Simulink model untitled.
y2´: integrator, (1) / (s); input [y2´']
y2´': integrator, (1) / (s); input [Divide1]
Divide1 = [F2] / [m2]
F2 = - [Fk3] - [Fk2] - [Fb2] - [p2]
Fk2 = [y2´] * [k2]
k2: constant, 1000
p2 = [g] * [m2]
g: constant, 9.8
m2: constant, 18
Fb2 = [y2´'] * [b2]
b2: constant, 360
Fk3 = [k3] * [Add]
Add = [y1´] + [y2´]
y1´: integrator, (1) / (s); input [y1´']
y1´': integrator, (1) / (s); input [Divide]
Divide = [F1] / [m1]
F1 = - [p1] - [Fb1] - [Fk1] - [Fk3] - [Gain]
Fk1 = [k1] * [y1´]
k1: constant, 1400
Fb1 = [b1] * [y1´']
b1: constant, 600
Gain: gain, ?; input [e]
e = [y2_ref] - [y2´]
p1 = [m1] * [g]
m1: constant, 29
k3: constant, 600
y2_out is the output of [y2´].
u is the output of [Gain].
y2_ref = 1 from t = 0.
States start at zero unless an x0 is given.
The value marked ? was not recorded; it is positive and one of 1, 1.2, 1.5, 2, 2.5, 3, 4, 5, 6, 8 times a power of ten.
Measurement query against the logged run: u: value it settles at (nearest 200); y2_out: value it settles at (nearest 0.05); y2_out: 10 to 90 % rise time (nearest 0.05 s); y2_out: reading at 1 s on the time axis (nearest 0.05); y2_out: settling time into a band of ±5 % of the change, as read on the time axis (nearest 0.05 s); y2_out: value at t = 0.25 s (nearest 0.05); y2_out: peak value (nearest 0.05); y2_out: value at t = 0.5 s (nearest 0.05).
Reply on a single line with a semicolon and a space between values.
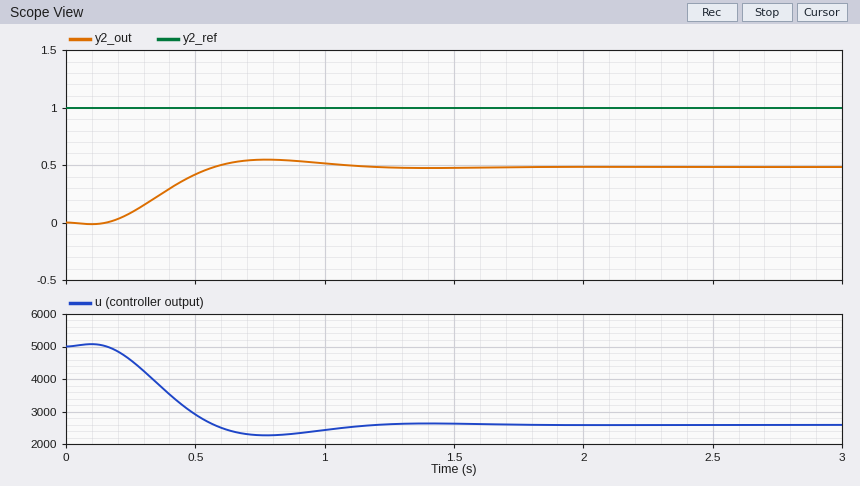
2600; 0.50; 0.30 s; 0.50; 1.05 s; 0.10; 0.55; 0.40
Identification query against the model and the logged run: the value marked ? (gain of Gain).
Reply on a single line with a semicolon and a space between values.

5000
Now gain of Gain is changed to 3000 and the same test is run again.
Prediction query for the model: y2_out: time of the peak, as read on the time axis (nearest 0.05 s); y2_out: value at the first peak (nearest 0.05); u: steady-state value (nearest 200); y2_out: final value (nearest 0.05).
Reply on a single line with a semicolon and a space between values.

0.95 s; 0.35; 2000; 0.35
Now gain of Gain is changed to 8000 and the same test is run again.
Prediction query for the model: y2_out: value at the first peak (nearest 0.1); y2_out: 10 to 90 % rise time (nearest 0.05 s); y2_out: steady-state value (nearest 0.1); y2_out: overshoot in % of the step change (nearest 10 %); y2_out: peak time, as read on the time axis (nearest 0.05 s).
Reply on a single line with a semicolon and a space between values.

0.8; 0.25 s; 0.6; 30 %; 0.65 s
